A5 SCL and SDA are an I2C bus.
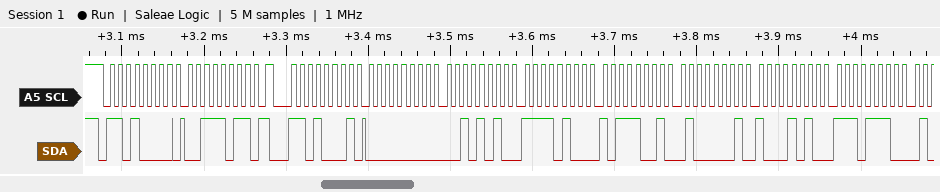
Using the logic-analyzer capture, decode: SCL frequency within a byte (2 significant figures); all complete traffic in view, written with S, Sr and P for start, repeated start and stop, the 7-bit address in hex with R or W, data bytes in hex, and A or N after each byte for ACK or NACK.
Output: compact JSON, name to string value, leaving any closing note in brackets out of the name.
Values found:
{"SCL frequency within a byte": "100 kHz", "all complete traffic in view, written with S, Sr and P for start, repeated start and stop, the 7-bit address in hex with R or W, data bytes in hex, and A or N after each byte for ACK or NACK": "S 68W A 3B A Sr 68R A 00 A 2A A F4 A B9 A 41 A 8A A EE A"}
